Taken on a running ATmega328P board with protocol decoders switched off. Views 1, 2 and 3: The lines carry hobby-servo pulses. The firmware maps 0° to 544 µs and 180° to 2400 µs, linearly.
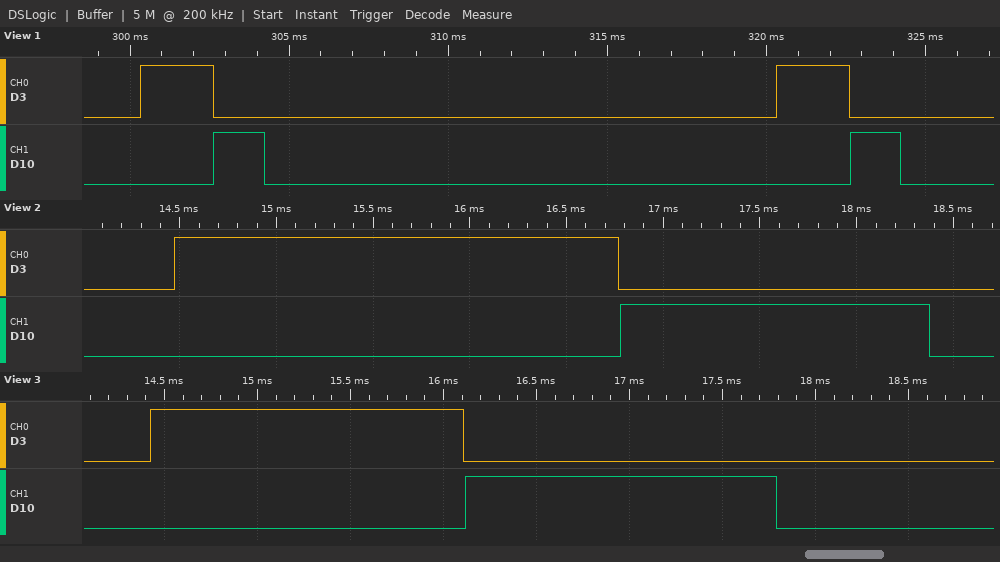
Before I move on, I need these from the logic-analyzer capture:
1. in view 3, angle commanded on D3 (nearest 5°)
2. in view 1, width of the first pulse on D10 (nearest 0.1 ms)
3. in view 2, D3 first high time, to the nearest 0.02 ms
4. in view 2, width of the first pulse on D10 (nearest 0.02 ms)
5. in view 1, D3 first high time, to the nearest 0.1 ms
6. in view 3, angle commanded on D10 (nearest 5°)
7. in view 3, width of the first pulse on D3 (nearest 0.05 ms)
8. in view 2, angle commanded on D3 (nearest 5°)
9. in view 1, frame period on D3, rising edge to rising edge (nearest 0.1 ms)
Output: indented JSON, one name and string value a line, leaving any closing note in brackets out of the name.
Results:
{
  "in view 3, angle commanded on D3": "110°",
  "in view 1, width of the first pulse on D10": "1.6 ms",
  "in view 2, D3 first high time, to the nearest 0.02 ms": "2.30 ms",
  "in view 2, width of the first pulse on D10": "1.60 ms",
  "in view 1, D3 first high time, to the nearest 0.1 ms": "2.3 ms",
  "in view 3, angle commanded on D10": "110°",
  "in view 3, width of the first pulse on D3": "1.70 ms",
  "in view 2, angle commanded on D3": "170°",
  "in view 1, frame period on D3, rising edge to rising edge": "20.0 ms"
}
